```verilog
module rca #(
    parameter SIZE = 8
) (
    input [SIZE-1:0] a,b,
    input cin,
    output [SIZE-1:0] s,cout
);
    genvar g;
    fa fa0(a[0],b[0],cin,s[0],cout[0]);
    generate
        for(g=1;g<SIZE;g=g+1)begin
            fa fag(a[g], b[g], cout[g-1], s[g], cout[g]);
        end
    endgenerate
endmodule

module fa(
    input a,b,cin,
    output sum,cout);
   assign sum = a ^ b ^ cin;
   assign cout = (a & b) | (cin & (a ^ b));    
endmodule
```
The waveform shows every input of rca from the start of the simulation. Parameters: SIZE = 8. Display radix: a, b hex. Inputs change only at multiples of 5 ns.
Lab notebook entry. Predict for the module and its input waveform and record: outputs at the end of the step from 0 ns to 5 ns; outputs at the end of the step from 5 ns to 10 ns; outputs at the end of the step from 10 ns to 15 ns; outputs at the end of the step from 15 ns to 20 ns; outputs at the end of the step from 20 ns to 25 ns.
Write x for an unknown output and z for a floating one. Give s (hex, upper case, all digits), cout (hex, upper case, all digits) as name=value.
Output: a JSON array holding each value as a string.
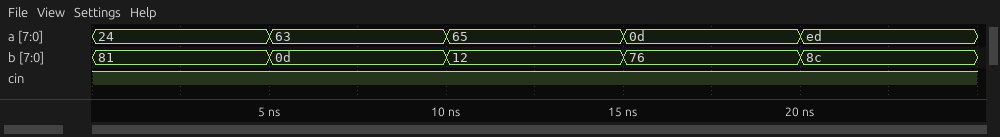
["s=A6, cout=01", "s=71, cout=0F", "s=78, cout=07", "s=84, cout=7F", "s=7A, cout=8D"]
